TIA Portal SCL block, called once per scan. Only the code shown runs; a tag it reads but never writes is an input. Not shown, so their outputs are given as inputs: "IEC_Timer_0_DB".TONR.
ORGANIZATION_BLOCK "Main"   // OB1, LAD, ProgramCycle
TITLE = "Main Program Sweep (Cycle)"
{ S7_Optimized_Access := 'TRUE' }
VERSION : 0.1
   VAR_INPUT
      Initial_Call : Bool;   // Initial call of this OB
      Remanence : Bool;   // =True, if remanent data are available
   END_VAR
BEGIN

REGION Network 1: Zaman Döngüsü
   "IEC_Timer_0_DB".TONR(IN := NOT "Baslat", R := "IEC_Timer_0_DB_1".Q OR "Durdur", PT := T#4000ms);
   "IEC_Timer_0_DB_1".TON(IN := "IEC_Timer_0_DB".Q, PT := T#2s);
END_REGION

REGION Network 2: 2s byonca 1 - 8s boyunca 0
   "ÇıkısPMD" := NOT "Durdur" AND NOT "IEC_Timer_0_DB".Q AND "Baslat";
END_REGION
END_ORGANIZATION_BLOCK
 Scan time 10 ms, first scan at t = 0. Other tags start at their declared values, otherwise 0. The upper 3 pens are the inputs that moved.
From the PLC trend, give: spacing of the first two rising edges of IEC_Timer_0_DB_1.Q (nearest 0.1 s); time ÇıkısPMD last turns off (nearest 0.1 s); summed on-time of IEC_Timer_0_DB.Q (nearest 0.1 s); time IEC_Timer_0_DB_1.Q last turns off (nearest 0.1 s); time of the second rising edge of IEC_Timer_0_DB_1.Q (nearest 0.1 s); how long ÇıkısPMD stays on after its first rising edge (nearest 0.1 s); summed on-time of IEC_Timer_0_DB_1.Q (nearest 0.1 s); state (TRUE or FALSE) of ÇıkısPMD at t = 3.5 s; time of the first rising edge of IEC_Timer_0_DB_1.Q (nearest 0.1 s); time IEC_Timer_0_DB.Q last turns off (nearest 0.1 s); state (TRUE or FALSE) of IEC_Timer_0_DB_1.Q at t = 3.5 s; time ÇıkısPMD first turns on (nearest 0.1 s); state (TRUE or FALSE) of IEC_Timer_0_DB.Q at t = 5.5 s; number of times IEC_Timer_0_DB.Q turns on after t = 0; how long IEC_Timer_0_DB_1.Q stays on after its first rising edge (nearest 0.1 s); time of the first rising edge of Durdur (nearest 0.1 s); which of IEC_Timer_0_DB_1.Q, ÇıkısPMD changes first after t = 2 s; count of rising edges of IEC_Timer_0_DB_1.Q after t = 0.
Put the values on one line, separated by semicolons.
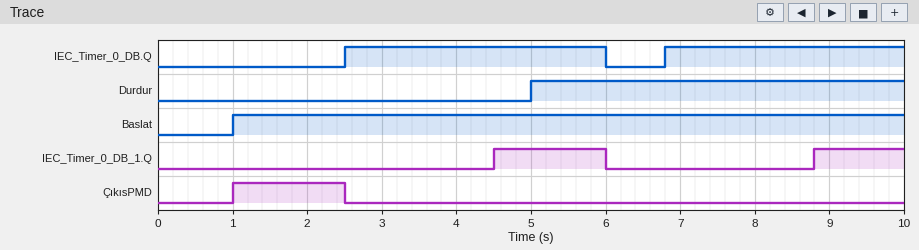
4.3 s; 2.5 s; 6.7 s; 6.0 s; 8.8 s; 1.5 s; 2.7 s; FALSE; 4.5 s; 6.0 s; FALSE; 1.0 s; TRUE; 2; 1.5 s; 5.0 s; ÇıkısPMD; 2
